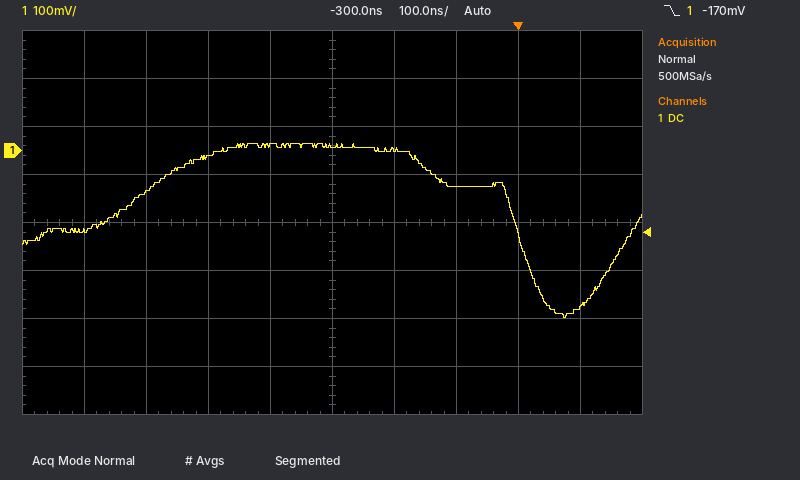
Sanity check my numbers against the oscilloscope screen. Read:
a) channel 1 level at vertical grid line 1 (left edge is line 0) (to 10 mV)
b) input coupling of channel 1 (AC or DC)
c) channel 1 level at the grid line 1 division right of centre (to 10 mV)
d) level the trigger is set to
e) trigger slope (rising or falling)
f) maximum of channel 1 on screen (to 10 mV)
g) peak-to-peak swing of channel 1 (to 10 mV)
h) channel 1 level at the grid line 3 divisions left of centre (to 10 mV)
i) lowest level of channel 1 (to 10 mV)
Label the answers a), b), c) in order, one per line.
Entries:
a) -170 mV
b) DC
c) 0 mV
d) -170 mV
e) falling
f) 10 mV
g) 360 mV
h) -90 mV
i) -350 mV
